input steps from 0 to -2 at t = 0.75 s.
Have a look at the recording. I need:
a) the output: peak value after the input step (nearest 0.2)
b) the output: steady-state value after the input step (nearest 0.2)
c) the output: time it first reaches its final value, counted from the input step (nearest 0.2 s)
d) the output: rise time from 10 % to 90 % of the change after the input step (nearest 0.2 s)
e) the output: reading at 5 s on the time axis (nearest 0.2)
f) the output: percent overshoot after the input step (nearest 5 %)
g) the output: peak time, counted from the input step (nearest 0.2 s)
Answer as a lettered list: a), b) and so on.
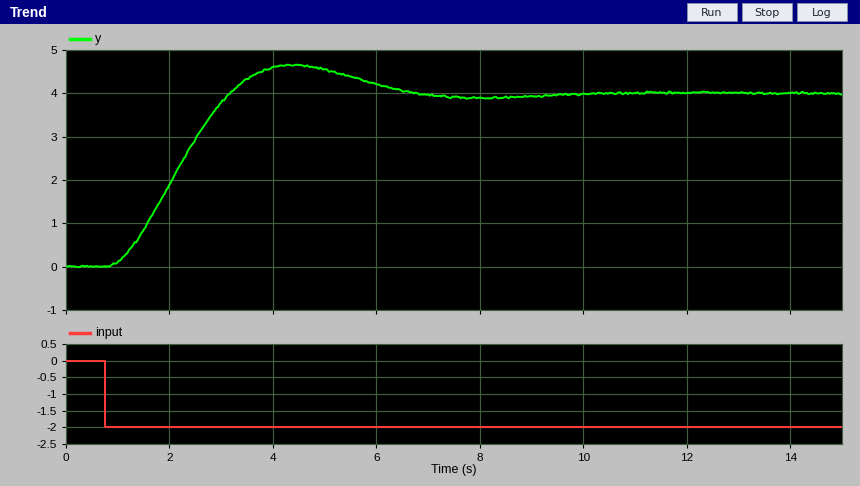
a) 4.6
b) 4.0
c) 2.4 s
d) 1.6 s
e) 4.6
f) 15 %
g) 3.6 s
